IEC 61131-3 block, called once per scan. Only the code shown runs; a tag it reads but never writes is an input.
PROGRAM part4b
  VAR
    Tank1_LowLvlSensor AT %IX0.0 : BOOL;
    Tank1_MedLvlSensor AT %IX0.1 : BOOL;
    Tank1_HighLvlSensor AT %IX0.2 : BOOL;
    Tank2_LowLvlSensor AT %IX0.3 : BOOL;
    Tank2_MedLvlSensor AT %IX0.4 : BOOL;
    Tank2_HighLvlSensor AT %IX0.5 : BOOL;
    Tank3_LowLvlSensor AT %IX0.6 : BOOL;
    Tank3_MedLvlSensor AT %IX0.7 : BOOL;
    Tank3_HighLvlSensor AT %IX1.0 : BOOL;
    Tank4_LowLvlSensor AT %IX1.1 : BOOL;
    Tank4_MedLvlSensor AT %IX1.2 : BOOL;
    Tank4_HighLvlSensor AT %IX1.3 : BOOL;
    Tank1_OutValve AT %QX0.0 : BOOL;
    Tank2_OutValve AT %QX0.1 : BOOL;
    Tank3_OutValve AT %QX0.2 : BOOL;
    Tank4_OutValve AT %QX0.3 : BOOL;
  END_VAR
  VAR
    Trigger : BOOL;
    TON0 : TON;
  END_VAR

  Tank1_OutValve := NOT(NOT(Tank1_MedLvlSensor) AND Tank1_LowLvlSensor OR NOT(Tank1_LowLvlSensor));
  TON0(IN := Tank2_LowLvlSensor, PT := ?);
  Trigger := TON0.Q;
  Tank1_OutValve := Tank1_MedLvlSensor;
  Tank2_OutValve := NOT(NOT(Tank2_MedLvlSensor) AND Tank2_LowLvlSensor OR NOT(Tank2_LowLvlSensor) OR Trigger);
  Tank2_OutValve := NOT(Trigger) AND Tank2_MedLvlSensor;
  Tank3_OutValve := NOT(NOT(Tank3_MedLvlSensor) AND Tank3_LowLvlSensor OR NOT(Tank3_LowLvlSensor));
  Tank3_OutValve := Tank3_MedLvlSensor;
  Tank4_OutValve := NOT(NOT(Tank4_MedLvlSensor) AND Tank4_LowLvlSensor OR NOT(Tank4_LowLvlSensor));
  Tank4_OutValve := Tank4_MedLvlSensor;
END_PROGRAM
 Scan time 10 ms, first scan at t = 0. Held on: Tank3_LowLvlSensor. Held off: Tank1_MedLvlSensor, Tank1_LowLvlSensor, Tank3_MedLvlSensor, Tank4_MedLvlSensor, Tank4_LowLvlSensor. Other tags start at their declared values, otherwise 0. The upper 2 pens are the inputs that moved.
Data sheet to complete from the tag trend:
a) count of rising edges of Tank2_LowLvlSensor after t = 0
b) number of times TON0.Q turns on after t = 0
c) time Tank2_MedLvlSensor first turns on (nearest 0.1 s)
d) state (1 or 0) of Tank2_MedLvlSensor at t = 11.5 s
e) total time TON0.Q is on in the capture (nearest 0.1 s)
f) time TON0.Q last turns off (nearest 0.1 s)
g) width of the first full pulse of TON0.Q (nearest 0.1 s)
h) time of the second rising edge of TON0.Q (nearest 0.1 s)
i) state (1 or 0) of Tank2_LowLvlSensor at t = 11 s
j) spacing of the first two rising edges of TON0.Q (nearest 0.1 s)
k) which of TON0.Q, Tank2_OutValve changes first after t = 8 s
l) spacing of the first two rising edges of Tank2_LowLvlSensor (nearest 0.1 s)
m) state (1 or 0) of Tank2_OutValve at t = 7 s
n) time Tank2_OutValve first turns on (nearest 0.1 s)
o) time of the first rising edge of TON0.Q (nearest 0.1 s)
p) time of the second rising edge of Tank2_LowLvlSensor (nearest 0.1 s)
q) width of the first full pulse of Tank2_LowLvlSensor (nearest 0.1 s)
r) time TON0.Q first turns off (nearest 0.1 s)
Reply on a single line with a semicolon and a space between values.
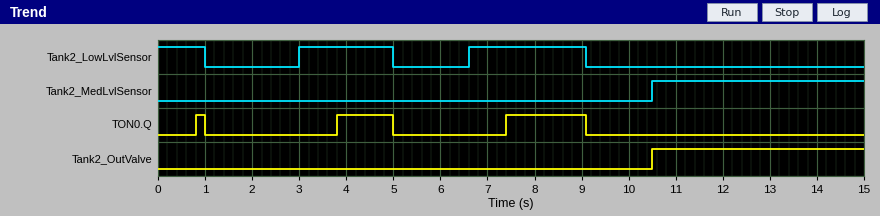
2; 3; 10.5 s; 1; 3.1 s; 9.1 s; 0.2 s; 3.8 s; 0; 3.0 s; TON0.Q; 3.6 s; 0; 10.5 s; 0.8 s; 6.6 s; 2.0 s; 1.0 s
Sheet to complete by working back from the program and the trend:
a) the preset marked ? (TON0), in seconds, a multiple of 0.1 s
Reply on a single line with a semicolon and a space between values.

0.8 s
